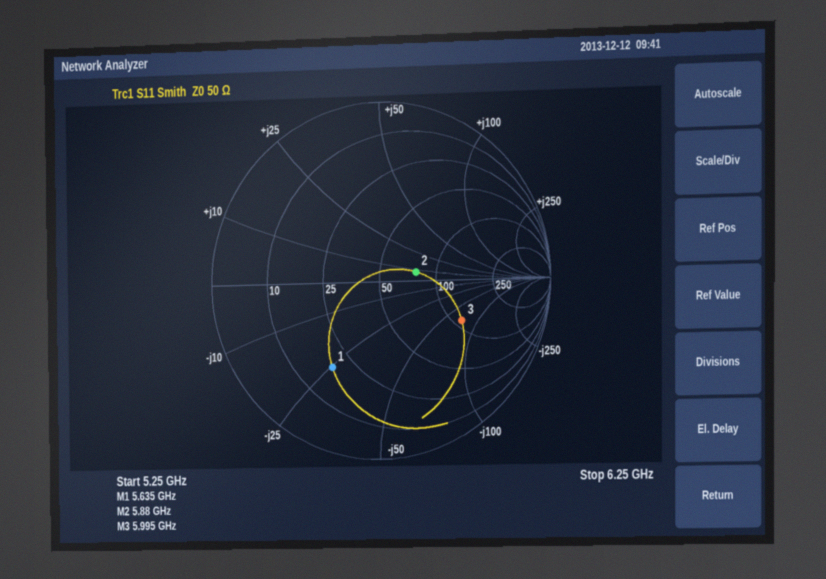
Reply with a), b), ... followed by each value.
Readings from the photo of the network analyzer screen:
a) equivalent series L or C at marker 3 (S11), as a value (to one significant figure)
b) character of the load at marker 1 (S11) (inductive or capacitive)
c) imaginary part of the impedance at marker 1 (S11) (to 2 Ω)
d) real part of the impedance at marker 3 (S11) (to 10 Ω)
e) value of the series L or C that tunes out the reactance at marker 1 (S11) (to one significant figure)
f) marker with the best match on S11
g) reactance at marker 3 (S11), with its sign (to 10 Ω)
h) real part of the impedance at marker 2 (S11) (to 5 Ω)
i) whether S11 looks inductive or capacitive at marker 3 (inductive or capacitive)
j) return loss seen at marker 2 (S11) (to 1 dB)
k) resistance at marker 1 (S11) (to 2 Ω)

a) 400 fF
b) capacitive
c) -26 Ω
d) 110 Ω
e) 700 pH
f) marker 2
g) -70 Ω
h) 75 Ω
i) capacitive
j) 13 dB
k) 18 Ω
